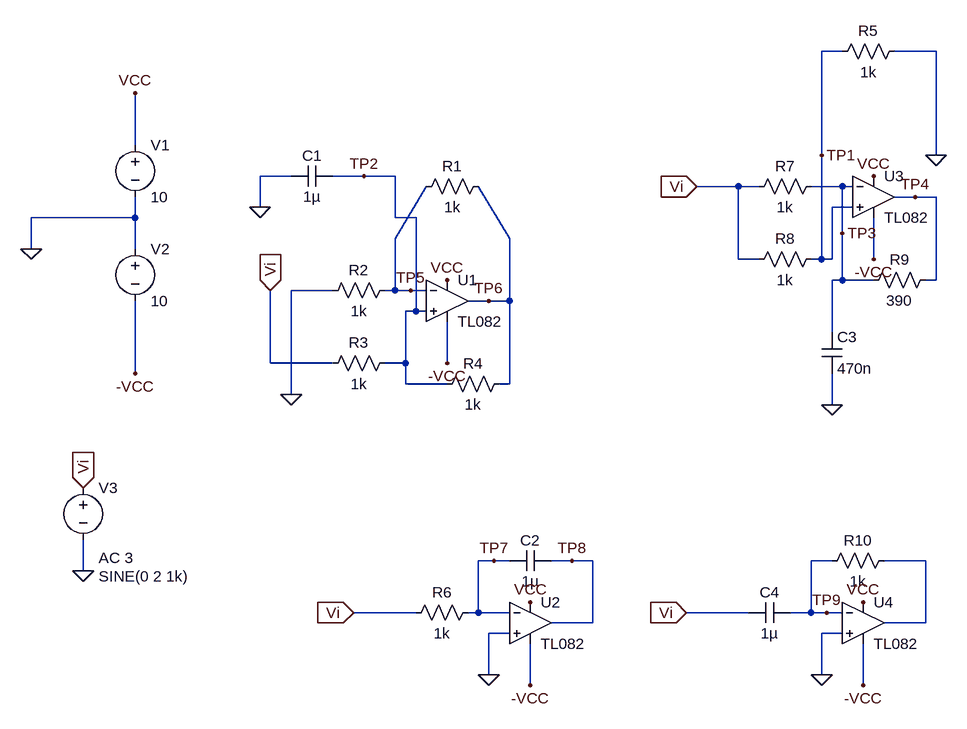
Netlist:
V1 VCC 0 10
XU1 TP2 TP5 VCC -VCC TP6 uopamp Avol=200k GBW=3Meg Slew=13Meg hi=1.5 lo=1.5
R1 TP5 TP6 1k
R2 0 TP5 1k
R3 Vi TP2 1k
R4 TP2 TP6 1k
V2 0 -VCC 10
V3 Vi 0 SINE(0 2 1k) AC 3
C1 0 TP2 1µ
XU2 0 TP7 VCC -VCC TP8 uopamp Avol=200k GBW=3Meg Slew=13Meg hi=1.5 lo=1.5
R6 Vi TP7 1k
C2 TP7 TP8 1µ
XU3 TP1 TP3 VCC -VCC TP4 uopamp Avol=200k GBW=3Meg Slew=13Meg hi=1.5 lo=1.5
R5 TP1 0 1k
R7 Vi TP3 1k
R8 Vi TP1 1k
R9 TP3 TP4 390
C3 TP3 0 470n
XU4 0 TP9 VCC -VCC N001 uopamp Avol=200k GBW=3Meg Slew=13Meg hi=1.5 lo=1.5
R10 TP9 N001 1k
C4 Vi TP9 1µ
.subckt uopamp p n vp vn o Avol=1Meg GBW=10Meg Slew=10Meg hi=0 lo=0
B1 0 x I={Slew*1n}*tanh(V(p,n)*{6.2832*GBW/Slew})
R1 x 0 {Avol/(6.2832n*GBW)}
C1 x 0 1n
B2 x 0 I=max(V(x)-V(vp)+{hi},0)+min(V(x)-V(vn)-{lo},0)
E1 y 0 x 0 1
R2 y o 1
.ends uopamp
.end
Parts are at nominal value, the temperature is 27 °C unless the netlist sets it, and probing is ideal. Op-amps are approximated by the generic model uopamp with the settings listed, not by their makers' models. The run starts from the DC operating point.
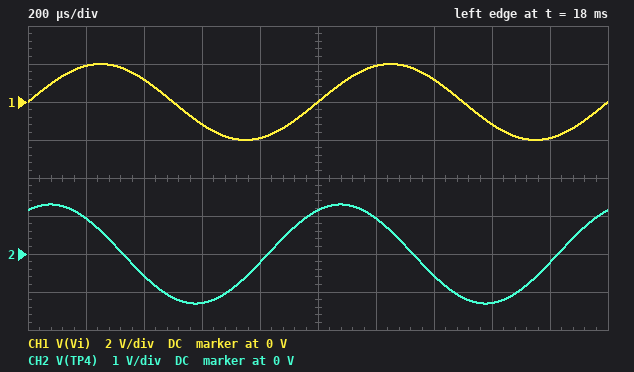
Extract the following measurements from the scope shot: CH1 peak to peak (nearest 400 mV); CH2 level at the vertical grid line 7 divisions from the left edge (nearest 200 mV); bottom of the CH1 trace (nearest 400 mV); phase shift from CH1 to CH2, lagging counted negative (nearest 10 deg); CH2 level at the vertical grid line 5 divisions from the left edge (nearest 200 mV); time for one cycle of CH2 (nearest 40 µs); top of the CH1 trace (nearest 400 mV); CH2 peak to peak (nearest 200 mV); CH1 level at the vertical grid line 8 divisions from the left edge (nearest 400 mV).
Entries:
4.0 V
-600 mV
-2.0 V
60 deg
1.2 V
1.00 ms
2.0 V
2.6 V
-1.2 V
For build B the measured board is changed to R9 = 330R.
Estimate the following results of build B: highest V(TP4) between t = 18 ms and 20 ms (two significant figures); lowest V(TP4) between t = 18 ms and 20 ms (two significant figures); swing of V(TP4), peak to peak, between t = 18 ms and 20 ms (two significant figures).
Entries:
1.2 V
-1.2 V
2.4 V
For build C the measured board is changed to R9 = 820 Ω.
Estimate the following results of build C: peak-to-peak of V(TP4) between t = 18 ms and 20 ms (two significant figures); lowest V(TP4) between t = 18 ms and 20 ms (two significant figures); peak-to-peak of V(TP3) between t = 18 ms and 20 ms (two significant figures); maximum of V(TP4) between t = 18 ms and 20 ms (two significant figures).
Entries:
4.9 V
-2.4 V
2.0 V
2.4 V
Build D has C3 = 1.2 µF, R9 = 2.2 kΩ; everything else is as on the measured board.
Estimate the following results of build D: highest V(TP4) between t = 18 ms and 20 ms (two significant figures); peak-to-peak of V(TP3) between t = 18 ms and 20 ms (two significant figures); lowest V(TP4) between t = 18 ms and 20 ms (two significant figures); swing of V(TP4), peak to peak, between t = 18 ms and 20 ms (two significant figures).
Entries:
8.5 V
1.9 V
-8.5 V
17 V
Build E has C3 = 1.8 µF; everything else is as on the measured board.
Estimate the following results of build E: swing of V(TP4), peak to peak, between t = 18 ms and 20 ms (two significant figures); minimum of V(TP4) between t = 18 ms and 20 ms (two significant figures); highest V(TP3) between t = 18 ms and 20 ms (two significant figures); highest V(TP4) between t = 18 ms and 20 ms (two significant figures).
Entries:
8.9 V
-4.5 V
1.0 V
4.5 V
